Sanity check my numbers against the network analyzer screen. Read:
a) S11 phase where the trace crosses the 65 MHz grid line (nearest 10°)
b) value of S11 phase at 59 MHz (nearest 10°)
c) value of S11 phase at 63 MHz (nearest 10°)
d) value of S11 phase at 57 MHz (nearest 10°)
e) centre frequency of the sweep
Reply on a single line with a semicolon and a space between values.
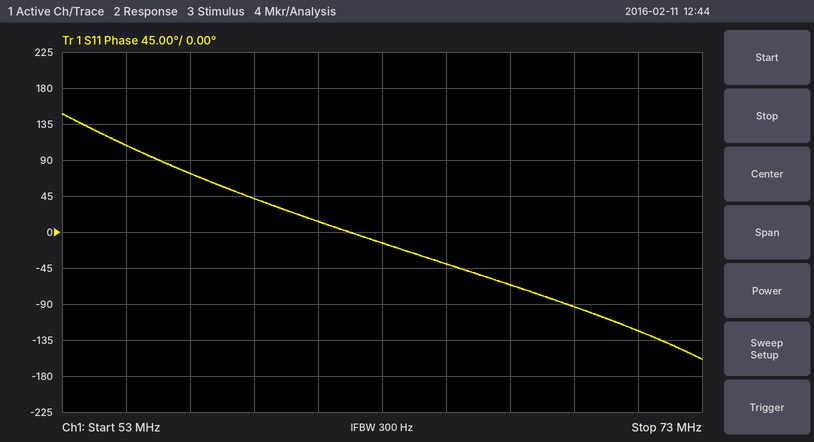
-40°; 40°; -10°; 70°; 63 MHz
